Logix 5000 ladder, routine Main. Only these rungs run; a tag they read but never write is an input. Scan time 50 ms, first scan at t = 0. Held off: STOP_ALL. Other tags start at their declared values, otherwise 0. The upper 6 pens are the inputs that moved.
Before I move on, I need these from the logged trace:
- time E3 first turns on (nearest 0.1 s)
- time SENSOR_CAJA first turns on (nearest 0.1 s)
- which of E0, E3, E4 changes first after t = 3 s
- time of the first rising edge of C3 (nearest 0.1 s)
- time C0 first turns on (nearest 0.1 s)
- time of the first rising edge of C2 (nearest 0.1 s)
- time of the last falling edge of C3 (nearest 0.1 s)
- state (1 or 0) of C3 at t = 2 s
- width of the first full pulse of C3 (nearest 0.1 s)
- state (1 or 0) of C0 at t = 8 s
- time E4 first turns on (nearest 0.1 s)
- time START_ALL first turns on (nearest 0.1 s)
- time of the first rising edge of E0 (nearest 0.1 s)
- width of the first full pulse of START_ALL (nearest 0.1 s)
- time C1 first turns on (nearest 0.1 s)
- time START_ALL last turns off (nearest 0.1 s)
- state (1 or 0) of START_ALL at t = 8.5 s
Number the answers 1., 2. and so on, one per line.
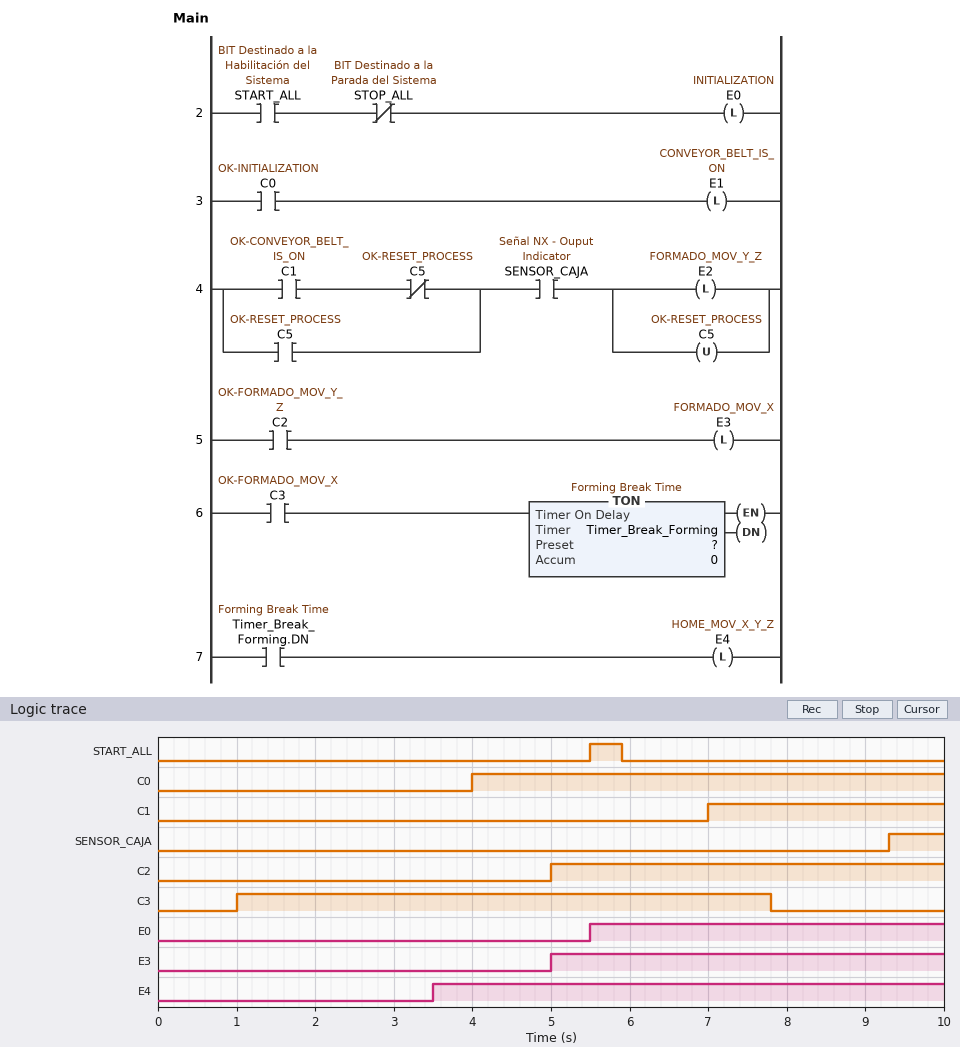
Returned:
1. 5.0 s
2. 9.3 s
3. E4
4. 1.0 s
5. 4.0 s
6. 5.0 s
7. 7.8 s
8. 1
9. 6.8 s
10. 1
11. 3.5 s
12. 5.5 s
13. 5.5 s
14. 0.4 s
15. 7.0 s
16. 5.9 s
17. 0
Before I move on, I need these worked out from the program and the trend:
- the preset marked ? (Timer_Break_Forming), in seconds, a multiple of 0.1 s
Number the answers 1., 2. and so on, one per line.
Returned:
1. 2.5 s
